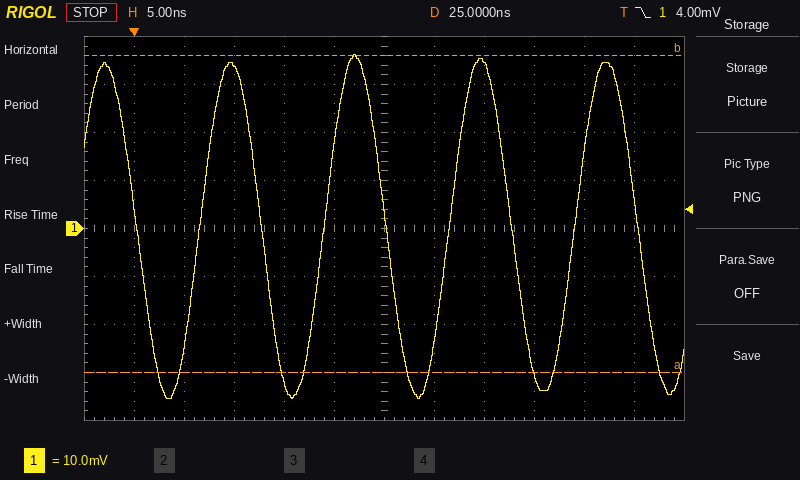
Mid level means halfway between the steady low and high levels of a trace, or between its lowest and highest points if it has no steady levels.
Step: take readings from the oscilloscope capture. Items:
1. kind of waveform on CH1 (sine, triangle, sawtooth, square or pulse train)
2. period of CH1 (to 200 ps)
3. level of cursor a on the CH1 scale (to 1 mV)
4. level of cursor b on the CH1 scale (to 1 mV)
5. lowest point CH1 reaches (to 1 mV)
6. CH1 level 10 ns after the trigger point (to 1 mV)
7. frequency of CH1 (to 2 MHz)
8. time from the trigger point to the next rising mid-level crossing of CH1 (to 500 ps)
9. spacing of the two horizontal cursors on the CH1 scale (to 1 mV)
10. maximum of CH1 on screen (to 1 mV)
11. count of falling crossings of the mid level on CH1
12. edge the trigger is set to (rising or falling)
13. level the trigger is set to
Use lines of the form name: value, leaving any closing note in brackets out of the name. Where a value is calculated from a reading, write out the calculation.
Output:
kind of waveform on CH1: sine
period of CH1: 12.6 ns
level of cursor a on the CH1 scale: -30 mV
level of cursor b on the CH1 scale: 36 mV
lowest point CH1 reaches: -35 mV
CH1 level 10 ns after the trigger point: 34 mV
frequency of CH1: 1 / 12.6 ns ≈ 79.4 MHz, so 80 MHz to the nearest 2 MHz
time from the trigger point to the next rising mid-level crossing of CH1: 6.5 ns
spacing of the two horizontal cursors on the CH1 scale: 66 mV
maximum of CH1 on screen: 36 mV
count of falling crossings of the mid level on CH1: 5
edge the trigger is set to: falling
level the trigger is set to: 4.00 mV
